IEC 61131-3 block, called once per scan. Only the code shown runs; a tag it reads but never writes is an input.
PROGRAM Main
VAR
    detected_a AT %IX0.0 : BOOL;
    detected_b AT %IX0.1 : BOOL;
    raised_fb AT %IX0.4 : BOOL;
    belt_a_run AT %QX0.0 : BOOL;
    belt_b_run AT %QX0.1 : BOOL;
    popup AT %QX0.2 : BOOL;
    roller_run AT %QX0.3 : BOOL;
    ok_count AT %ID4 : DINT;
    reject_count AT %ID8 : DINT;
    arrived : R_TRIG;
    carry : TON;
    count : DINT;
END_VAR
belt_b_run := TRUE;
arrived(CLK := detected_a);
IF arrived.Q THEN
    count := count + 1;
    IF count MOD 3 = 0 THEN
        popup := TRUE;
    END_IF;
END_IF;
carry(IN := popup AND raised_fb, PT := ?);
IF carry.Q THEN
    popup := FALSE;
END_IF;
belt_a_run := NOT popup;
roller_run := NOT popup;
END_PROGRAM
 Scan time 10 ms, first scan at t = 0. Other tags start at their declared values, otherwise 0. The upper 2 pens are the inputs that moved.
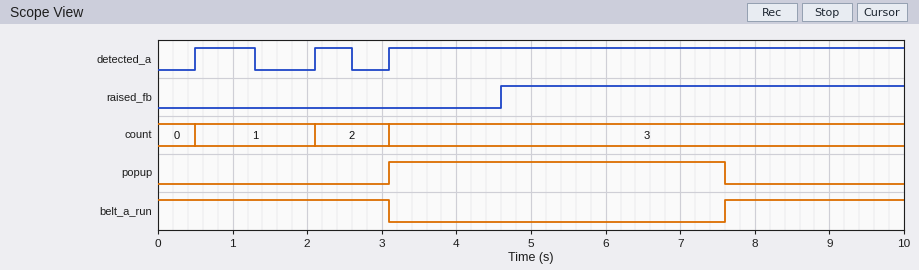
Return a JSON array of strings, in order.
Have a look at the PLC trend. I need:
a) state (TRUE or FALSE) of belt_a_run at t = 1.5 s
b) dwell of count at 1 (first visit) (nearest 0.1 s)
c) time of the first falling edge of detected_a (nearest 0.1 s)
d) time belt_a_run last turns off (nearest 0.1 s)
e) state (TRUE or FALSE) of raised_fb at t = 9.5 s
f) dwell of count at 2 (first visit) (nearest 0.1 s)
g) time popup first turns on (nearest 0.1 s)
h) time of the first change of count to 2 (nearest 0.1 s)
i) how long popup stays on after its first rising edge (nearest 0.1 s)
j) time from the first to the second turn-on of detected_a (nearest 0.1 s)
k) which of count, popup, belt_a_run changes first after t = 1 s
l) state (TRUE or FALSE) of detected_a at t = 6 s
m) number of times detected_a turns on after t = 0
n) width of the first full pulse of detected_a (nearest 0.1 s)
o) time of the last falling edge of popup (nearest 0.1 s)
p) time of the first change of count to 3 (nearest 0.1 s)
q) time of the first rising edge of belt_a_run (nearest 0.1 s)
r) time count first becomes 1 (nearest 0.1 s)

["TRUE", "1.6 s", "1.3 s", "3.1 s", "TRUE", "1.0 s", "3.1 s", "2.1 s", "4.5 s", "1.6 s", "count", "TRUE", "3", "0.8 s", "7.6 s", "3.1 s", "7.6 s", "0.5 s"]
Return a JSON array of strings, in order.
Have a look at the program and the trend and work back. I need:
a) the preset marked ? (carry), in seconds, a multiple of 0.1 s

["3.0 s"]
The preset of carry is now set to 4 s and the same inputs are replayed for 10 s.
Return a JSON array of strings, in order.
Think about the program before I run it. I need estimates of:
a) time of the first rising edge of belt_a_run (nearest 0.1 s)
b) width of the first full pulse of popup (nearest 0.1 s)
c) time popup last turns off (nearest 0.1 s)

["8.6 s", "5.5 s", "8.6 s"]
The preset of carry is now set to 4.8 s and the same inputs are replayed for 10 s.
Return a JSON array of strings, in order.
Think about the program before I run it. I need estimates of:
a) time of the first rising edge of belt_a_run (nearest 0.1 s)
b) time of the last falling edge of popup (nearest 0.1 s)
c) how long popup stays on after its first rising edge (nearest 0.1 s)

["9.4 s", "9.4 s", "6.3 s"]
